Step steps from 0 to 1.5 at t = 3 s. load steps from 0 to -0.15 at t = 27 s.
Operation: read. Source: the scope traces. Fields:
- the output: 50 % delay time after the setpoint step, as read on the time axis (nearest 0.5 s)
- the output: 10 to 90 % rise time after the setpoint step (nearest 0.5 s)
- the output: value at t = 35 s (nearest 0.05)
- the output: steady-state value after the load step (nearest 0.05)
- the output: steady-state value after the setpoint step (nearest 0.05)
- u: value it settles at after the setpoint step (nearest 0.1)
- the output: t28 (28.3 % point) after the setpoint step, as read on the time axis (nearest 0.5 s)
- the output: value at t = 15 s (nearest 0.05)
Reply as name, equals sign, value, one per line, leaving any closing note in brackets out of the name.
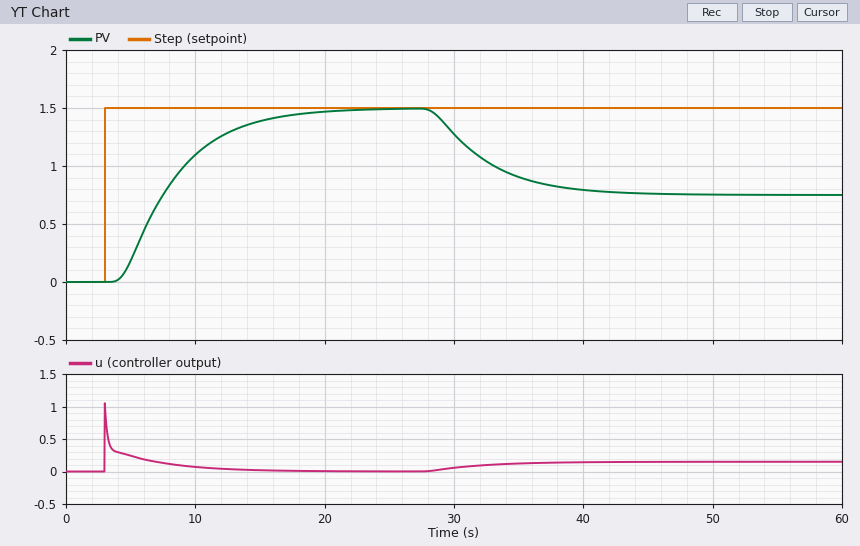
the output: 50 % delay time after the setpoint step, as read on the time axis = 7.5 s
the output: 10 to 90 % rise time after the setpoint step = 9.0 s
the output: value at t = 35 s = 0.90
the output: steady-state value after the load step = 0.75
the output: steady-state value after the setpoint step = 1.50
u: value it settles at after the setpoint step = 0.0
the output: t28 (28.3 % point) after the setpoint step, as read on the time axis = 6.0 s
the output: value at t = 15 s = 1.40
